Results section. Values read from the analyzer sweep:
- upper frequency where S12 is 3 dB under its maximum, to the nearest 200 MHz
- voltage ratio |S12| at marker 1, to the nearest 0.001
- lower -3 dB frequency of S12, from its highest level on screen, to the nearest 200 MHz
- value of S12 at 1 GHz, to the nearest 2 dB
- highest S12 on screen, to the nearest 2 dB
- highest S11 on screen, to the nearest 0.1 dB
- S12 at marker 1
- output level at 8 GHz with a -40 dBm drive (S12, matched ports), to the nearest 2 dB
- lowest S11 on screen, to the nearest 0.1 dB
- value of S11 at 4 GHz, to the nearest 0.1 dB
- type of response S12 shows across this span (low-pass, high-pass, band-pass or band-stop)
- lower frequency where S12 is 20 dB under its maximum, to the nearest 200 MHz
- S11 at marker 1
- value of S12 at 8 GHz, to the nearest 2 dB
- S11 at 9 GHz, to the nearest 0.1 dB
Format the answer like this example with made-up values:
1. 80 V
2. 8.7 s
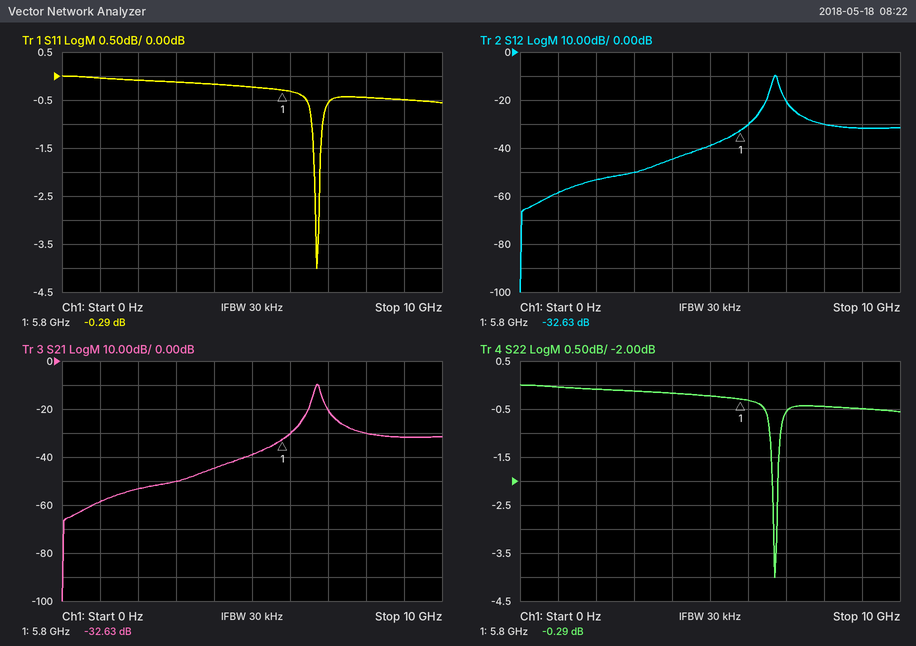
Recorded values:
1. 6.8 GHz
2. 0.023
3. 6.6 GHz
4. -58 dB
5. -10 dB
6. 0.0 dB
7. -32.63 dB
8. -70 dBm
9. -4.0 dB
10. -0.2 dB
11. band-pass
12. 6.0 GHz
13. -0.29 dB
14. -30 dB
15. -0.5 dB
